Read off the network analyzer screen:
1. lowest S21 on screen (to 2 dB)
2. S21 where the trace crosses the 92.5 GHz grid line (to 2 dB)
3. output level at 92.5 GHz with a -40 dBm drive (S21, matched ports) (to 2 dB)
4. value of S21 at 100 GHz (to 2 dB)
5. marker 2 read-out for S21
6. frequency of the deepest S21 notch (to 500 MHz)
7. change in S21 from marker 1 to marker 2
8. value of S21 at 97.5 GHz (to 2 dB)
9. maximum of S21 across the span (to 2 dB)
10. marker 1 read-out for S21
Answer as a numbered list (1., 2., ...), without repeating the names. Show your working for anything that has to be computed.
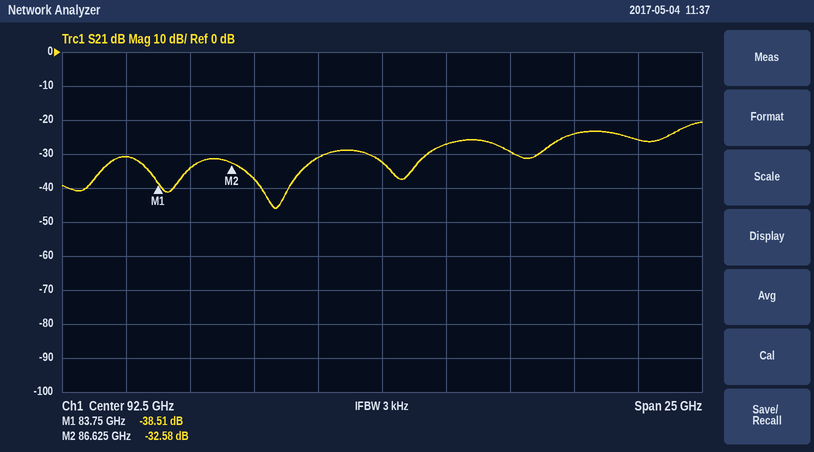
1. -46 dB
2. -32 dB
3. -40 dBm + (-32 dB) = -72 dBm
4. -24 dB
5. -32.58 dB
6. 88.5 GHz
7. -32.58 − (-38.51) = 5.93 dB
8. -30 dB
9. -20 dB
10. -38.51 dB
